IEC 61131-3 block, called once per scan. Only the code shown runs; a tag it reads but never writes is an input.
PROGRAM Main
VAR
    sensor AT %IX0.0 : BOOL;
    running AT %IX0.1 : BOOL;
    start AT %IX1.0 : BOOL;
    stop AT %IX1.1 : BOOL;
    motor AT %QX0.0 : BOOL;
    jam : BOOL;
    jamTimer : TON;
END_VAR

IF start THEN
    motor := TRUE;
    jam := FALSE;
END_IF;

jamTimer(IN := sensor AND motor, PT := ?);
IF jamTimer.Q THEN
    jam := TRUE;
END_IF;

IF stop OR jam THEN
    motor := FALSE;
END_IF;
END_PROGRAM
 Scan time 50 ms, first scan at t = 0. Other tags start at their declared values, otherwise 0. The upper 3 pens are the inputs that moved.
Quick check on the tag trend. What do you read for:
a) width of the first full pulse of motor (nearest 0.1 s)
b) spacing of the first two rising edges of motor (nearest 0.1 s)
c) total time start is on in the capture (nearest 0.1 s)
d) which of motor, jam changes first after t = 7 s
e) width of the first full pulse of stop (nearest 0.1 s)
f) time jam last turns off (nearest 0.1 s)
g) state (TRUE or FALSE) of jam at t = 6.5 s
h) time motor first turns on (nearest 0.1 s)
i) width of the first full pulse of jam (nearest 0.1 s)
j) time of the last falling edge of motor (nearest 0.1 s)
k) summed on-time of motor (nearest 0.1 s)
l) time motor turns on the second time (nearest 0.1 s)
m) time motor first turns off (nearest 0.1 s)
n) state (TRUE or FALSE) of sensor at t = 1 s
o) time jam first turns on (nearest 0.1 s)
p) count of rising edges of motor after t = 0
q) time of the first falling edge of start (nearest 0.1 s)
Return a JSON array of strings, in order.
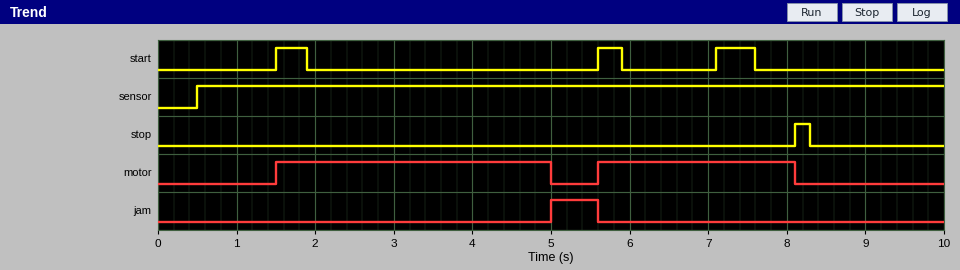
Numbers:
["3.5 s", "4.1 s", "1.2 s", "motor", "0.2 s", "5.6 s", "FALSE", "1.5 s", "0.6 s", "8.1 s", "6.0 s", "5.6 s", "5.0 s", "TRUE", "5.0 s", "2", "1.9 s"]
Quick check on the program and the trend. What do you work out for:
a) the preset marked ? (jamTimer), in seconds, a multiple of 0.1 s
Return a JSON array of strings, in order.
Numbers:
["3.5 s"]
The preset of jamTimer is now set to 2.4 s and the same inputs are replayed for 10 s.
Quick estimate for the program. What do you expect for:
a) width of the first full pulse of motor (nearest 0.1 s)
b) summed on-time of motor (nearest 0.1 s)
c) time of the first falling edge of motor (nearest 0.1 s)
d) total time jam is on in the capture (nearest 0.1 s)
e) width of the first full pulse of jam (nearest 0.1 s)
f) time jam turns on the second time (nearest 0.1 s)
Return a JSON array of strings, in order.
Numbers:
["2.4 s", "4.8 s", "3.9 s", "3.7 s", "1.7 s", "8.0 s"]
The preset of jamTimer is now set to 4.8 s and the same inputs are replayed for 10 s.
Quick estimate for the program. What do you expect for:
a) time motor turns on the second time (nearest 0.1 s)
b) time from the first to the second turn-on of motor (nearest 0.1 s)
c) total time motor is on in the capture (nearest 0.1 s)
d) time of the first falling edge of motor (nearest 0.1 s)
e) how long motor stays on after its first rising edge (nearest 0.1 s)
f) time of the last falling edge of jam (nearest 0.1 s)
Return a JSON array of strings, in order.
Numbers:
["7.1 s", "5.6 s", "5.8 s", "6.3 s", "4.8 s", "7.1 s"]
